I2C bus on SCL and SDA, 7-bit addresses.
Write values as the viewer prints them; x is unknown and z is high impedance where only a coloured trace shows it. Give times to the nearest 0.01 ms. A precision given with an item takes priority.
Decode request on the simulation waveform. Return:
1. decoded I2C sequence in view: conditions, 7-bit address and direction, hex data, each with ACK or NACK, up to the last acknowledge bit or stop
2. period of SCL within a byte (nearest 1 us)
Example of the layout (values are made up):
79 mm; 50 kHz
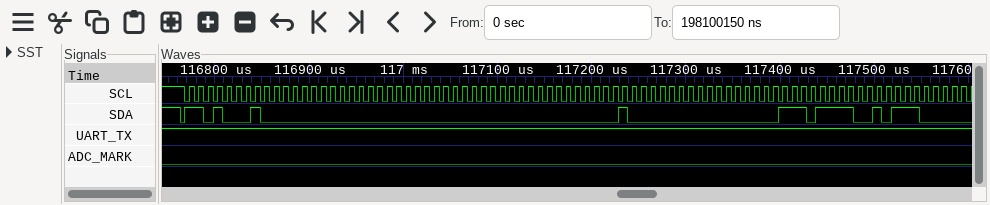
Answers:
start, address 68 read ACK, 00 ACK, 00 ACK, 00 ACK, 00 ACK, 40 ACK, 00 ACK, EF ACK, 5C ACK; 10 us
